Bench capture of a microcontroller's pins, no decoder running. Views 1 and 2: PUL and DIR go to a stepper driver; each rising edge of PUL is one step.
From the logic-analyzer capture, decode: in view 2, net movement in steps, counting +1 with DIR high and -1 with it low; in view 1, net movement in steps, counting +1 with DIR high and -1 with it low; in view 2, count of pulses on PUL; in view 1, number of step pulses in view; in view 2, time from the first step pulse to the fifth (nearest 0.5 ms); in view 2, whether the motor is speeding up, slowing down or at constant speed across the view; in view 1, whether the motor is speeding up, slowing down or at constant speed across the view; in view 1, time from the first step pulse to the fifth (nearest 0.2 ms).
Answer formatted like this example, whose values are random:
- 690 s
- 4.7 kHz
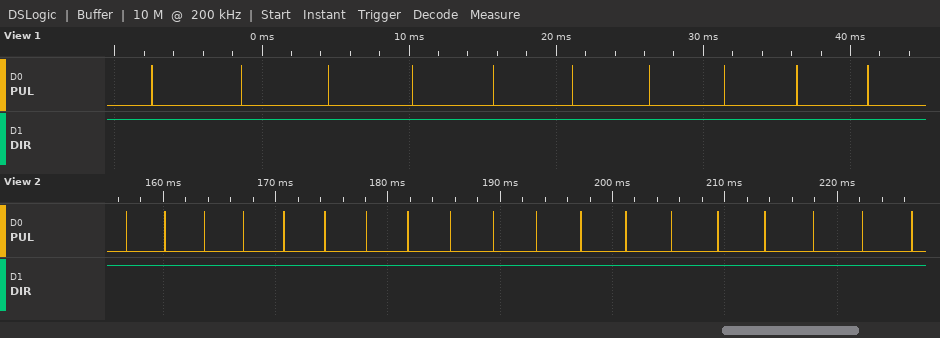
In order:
- +19
- +10
- 19
- 10
- 14.0 ms
- slowing down
- speeding up
- 23.2 ms
